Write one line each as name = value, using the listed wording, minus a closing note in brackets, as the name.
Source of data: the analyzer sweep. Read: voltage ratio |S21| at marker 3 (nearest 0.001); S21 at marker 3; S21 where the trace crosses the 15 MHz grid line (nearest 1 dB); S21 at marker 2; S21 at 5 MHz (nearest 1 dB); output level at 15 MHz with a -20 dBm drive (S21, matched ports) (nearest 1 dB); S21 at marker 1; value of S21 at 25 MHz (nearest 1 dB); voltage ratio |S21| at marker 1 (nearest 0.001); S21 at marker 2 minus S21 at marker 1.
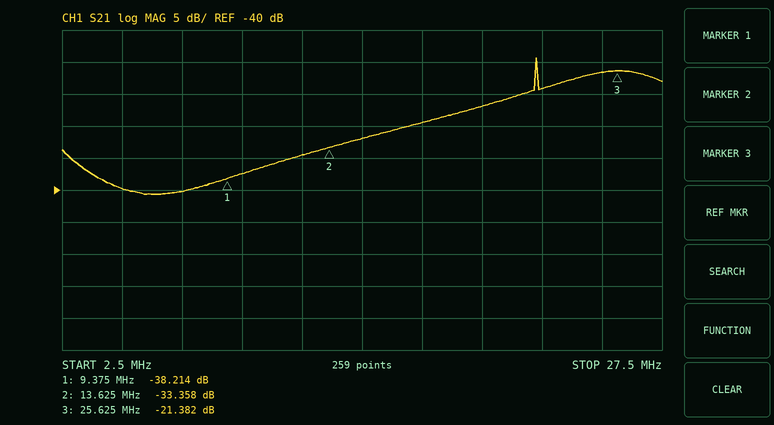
voltage ratio |S21| at marker 3 = 0.085
S21 at marker 3 = -21.382 dB
S21 where the trace crosses the 15 MHz grid line = -32 dB
S21 at marker 2 = -33.358 dB
S21 at 5 MHz = -40 dB
output level at 15 MHz with a -20 dBm drive (S21, matched ports) = -52 dBm
S21 at marker 1 = -38.214 dB
value of S21 at 25 MHz = -22 dB
voltage ratio |S21| at marker 1 = 0.012
S21 at marker 2 minus S21 at marker 1 = 4.856 dB
